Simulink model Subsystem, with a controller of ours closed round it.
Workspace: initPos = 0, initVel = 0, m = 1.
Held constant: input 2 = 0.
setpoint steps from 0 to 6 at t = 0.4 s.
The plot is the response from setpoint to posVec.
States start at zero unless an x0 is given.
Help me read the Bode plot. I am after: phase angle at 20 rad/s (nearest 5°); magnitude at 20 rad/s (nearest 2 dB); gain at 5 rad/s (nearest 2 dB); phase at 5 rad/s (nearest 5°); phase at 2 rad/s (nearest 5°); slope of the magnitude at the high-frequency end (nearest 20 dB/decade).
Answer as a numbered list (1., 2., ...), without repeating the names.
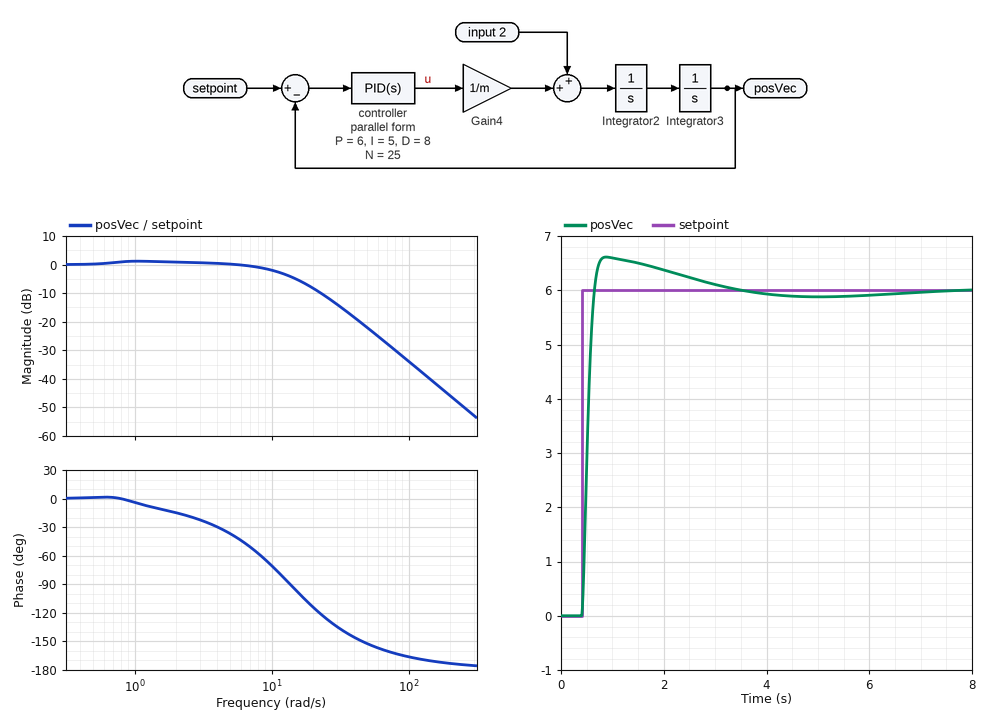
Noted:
1. -115°
2. -8 dB
3. 0 dB
4. -35°
5. -15°
6. -40 dB/decade
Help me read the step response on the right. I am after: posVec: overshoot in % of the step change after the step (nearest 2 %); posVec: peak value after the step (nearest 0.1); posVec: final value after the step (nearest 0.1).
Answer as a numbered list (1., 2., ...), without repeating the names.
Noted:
1. 10 %
2. 6.6
3. 6.0
